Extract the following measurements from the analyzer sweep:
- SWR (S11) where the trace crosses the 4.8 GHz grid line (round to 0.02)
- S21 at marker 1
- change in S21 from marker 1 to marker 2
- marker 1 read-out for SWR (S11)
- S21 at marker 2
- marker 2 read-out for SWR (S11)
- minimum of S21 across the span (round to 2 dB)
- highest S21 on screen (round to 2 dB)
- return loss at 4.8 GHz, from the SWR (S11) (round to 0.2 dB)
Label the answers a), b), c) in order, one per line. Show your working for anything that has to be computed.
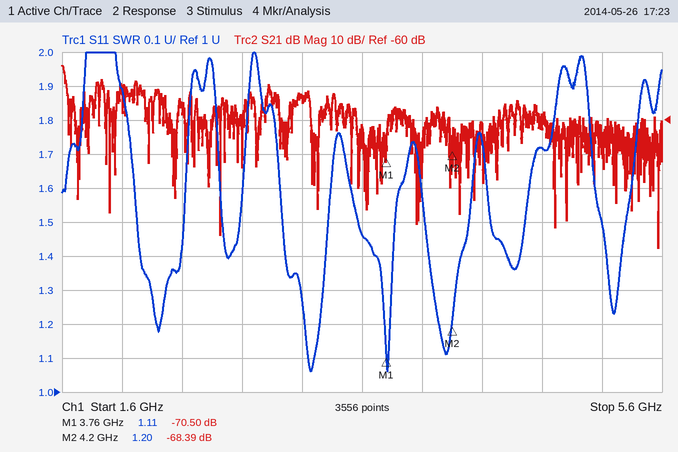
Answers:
a) 1.72
b) -70.50 dB
c) -68.39 − (-70.5) = 2.11 dB
d) 1.11
e) -68.39 dB
f) 1.20
g) -98 dB
h) -44 dB
i) −20 log10((1.72 − 1)/(1.72 + 1)) ≈ 11.5 dB, so 11.6 dB to the nearest 0.2 dB
